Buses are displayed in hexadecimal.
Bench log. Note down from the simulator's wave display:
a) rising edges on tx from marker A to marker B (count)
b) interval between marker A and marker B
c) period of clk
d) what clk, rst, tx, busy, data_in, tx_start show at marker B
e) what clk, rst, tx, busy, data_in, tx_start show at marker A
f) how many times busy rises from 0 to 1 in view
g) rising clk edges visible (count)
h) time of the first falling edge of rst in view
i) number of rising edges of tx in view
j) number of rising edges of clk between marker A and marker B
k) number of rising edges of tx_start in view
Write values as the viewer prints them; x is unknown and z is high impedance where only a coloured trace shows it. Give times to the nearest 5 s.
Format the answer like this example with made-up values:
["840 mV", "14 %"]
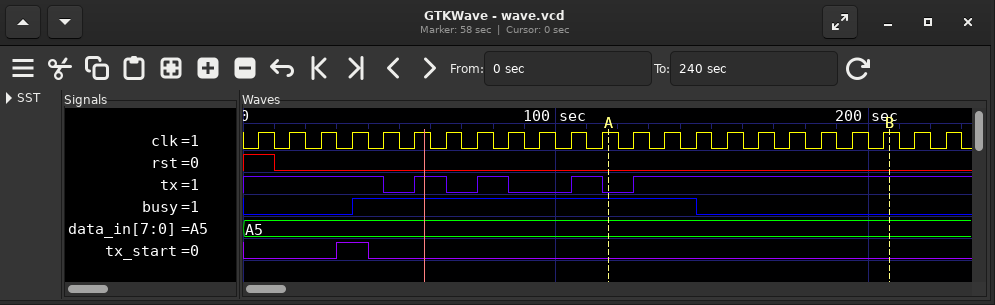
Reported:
["1", "90 s", "10 s", "clk=1, rst=0, tx=1, busy=0, data_in=A5, tx_start=0", "clk=1, rst=0, tx=0, busy=1, data_in=A5, tx_start=0", "1", "23", "10 s", "4", "9", "1"]
